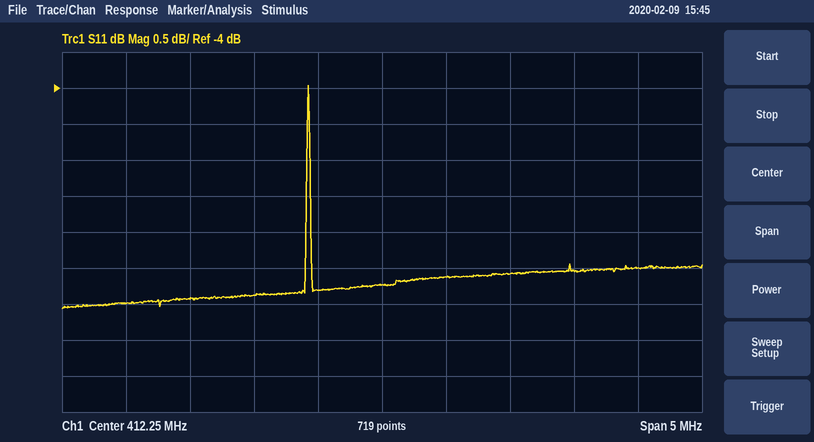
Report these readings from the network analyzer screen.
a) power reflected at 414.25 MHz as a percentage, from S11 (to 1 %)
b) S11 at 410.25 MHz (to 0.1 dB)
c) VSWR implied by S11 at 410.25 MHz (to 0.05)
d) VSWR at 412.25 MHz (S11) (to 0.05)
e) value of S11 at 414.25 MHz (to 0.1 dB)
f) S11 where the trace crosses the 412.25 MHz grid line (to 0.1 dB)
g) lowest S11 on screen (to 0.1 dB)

22 %
-7.0 dB
2.60
2.70
-6.5 dB
-6.7 dB
-7.1 dB
